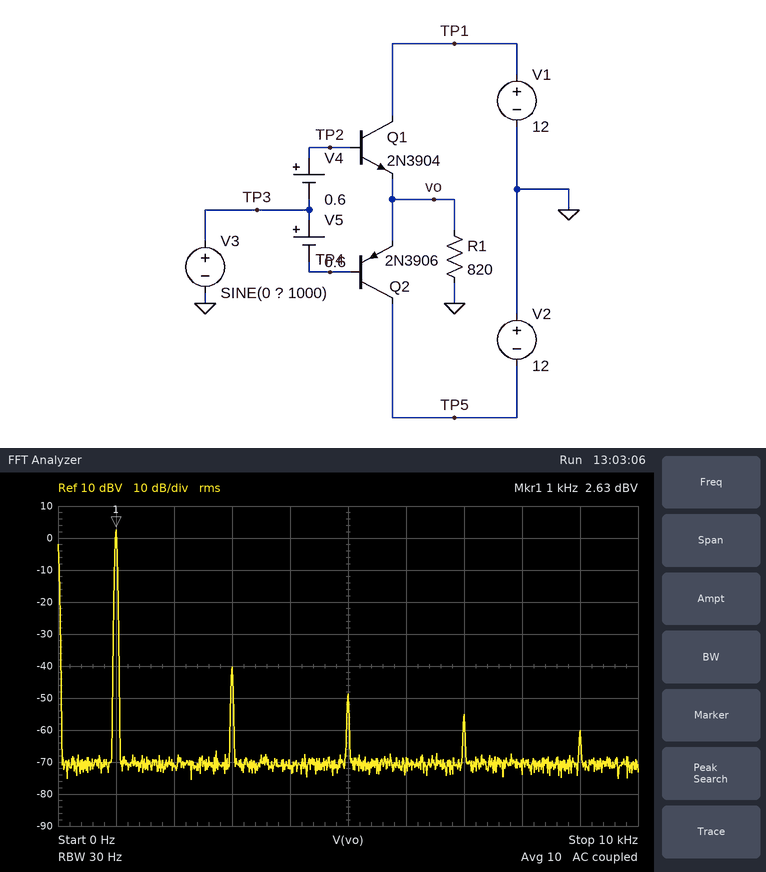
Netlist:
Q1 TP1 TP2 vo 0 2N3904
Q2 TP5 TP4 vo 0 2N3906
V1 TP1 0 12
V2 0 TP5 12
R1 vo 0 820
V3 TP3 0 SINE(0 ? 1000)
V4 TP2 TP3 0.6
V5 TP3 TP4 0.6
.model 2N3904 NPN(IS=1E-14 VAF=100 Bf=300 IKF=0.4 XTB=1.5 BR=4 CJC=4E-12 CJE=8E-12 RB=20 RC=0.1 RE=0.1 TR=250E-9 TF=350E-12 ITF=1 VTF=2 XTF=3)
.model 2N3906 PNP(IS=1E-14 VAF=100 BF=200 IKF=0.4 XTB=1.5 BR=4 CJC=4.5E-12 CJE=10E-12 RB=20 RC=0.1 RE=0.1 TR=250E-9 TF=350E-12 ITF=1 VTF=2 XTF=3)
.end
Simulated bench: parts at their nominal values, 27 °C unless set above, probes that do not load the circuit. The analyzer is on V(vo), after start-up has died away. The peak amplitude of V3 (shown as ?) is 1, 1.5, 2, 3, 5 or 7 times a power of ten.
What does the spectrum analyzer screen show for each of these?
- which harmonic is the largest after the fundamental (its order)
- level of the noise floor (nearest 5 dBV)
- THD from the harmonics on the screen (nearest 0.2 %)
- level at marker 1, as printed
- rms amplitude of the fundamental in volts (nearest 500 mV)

3
-70 dBV
0.8 %
2.63 dBV
1.5 V
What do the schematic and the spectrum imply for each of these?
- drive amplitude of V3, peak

2 V
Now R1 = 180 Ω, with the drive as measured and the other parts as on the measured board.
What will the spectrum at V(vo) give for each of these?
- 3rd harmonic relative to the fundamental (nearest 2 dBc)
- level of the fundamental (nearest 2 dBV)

-36 dBc
2 dBV
